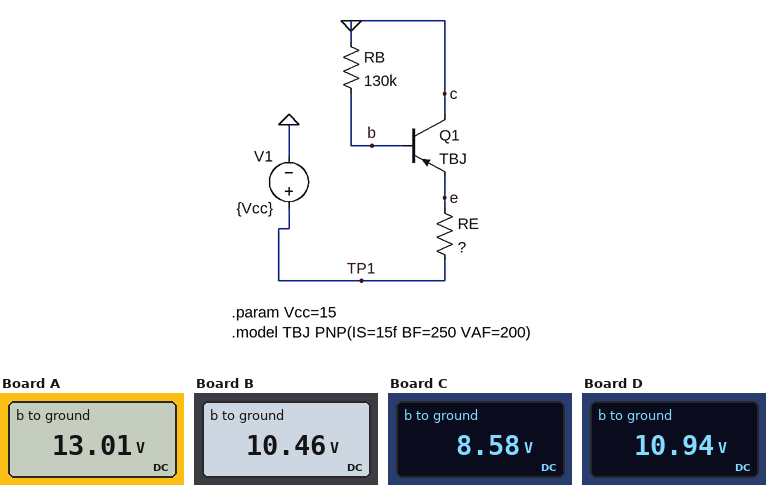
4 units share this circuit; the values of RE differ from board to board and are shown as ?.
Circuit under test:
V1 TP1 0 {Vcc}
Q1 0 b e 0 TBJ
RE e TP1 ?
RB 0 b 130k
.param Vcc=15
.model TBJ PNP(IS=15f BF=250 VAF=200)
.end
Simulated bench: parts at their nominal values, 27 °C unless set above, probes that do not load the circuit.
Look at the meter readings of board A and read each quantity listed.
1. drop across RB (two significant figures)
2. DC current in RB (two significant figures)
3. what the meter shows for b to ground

13 V
100 µA
13.01 V
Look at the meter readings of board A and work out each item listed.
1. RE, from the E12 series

47 Ω
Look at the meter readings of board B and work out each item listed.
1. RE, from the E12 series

180 Ω
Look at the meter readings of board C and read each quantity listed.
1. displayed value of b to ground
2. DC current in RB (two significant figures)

8.58 V
66 µA
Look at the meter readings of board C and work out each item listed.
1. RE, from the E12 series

330 Ω
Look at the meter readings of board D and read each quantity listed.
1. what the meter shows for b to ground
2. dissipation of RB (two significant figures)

10.94 V
920 µW
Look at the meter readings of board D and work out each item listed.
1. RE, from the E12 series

150 Ω
